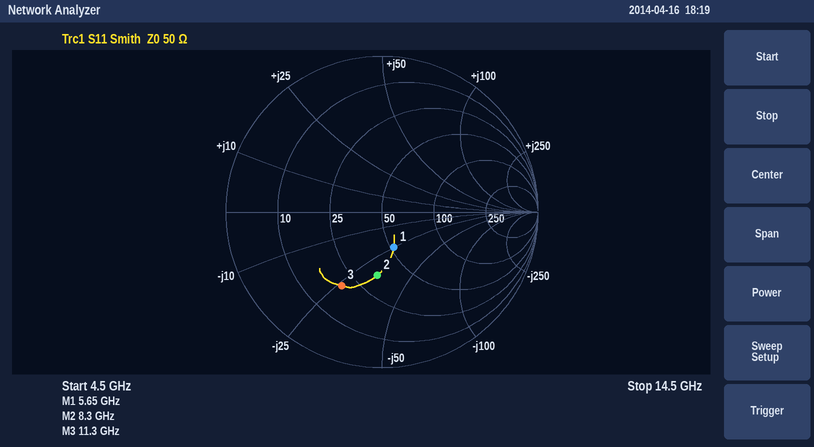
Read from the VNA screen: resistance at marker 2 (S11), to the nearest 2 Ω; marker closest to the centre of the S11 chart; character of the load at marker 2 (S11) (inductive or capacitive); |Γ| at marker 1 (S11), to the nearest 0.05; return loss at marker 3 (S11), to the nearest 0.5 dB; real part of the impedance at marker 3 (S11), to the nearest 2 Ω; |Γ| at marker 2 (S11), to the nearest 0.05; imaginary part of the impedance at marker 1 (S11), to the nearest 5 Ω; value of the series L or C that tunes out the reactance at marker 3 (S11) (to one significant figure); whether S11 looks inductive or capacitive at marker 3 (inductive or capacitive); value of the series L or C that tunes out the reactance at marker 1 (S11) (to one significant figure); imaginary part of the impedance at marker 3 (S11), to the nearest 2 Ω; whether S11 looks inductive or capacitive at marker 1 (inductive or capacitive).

34 Ω
marker 1
capacitive
0.25
5.5 dB
20 Ω
0.40
-25 Ω
400 pH
capacitive
700 pH
-26 Ω
capacitive
